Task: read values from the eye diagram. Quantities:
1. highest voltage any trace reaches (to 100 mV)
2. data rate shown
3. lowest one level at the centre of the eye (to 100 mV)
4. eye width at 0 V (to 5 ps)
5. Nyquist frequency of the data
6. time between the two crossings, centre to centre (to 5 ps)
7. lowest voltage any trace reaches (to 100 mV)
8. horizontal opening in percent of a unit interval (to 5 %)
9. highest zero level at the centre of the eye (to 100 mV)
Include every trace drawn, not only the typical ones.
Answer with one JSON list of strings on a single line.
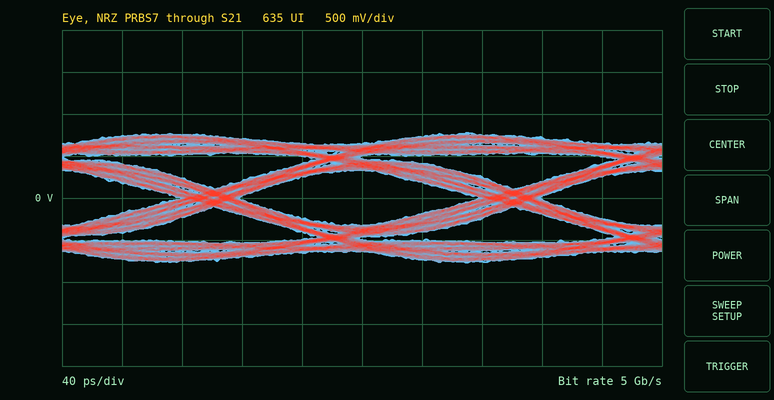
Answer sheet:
["800 mV", "5 Gb/s", "300 mV", "160 ps", "2.5 GHz", "200 ps", "-800 mV", "80 %", "-300 mV"]
